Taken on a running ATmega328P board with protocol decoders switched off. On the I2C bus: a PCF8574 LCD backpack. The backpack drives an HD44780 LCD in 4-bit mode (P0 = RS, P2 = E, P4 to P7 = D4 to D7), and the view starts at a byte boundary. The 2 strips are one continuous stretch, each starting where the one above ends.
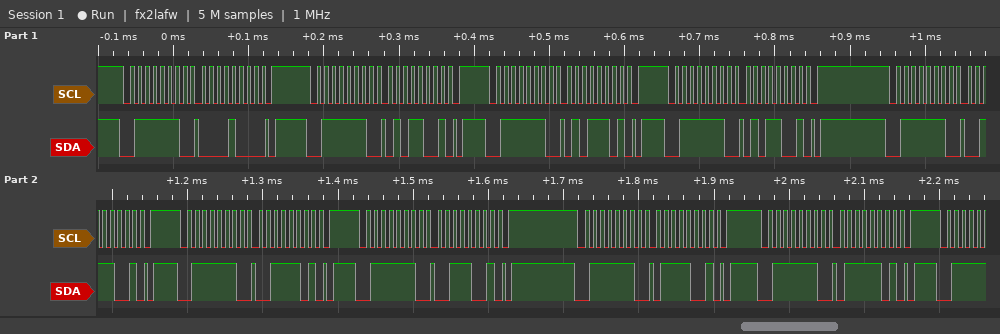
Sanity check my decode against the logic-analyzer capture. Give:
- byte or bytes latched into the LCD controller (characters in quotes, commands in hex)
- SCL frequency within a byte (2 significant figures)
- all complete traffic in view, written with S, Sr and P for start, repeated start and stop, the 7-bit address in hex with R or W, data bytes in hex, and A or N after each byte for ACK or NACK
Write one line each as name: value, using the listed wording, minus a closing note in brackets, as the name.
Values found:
byte or bytes latched into the LCD controller: 'S'
SCL frequency within a byte: 100 kHz
all complete traffic in view, written with S, Sr and P for start, repeated start and stop, the 7-bit address in hex with R or W, data bytes in hex, and A or N after each byte for ACK or NACK: S 3FW A 08 A P S 3FW A 59 A P S 3FW A 5D A P S 3FW A 59 A P S 3FW A 39 A P S 3FW A 3D A P S 3FW A 39 A P S 3FW A 79 A P S 3FW A 7D A P
